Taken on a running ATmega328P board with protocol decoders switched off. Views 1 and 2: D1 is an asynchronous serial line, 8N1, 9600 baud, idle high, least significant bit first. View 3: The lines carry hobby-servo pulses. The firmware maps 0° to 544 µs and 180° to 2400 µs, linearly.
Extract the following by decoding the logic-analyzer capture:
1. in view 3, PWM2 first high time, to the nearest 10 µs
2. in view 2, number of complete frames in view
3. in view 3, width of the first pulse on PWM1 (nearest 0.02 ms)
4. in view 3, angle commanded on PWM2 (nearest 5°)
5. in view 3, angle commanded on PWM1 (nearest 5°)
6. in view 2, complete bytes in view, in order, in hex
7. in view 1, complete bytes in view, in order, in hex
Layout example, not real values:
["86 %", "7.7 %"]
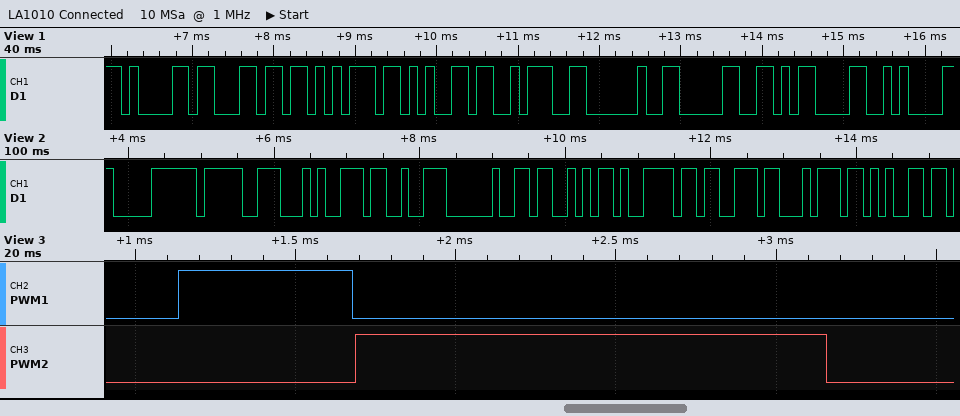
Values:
["1470 µs", "10", "0.54 ms", "90°", "0°", "F0 9F 94 93 20 53 79 73 74 65", "0x61 0x6C 0x75 0x65 0x3A 0x20 0x30 0x0D 0x0A"]
